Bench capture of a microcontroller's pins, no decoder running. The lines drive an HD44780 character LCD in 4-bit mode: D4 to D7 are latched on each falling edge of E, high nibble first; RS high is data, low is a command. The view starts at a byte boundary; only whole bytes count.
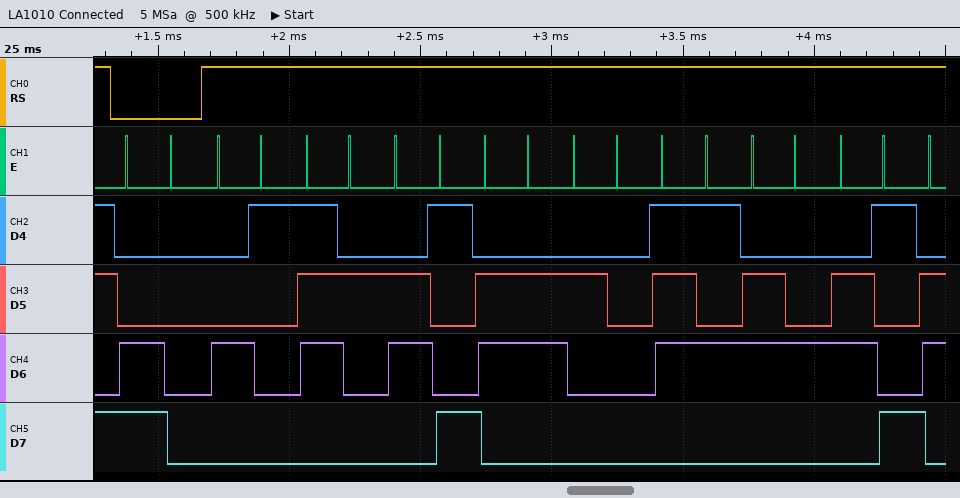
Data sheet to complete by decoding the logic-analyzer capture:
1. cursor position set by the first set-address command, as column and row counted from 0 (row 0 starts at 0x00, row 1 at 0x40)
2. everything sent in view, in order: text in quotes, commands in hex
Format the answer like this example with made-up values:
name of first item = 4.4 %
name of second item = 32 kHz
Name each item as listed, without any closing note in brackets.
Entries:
cursor position set by the first set-address command, as column and row counted from 0 = column 0, row 1
everything sent in view, in order: text in quotes, commands in hex = 0xC0 "Arif udi"
